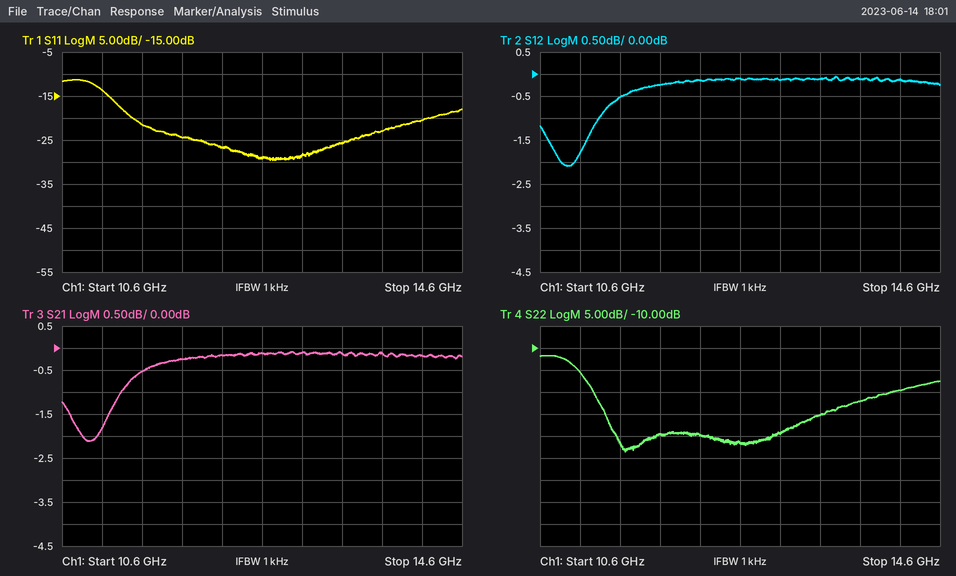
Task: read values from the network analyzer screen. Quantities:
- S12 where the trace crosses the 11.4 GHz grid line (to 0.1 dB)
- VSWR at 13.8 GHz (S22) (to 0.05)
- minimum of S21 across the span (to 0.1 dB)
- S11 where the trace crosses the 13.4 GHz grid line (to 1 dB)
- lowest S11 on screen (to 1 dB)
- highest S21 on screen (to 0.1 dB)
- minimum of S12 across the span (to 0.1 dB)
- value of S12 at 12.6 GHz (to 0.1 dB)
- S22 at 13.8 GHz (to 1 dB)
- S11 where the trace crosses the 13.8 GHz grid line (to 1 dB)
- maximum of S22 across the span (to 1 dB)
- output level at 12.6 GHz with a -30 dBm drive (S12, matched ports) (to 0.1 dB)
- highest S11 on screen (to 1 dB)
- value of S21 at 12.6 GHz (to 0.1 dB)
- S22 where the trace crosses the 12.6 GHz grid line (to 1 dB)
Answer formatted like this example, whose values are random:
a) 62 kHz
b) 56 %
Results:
a) -0.5 dB
b) 1.15
c) -2.1 dB
d) -26 dB
e) -30 dB
f) -0.1 dB
g) -2.1 dB
h) -0.1 dB
i) -22 dB
j) -23 dB
k) -12 dB
l) -30.1 dBm
m) -11 dB
n) -0.1 dB
o) -32 dB
